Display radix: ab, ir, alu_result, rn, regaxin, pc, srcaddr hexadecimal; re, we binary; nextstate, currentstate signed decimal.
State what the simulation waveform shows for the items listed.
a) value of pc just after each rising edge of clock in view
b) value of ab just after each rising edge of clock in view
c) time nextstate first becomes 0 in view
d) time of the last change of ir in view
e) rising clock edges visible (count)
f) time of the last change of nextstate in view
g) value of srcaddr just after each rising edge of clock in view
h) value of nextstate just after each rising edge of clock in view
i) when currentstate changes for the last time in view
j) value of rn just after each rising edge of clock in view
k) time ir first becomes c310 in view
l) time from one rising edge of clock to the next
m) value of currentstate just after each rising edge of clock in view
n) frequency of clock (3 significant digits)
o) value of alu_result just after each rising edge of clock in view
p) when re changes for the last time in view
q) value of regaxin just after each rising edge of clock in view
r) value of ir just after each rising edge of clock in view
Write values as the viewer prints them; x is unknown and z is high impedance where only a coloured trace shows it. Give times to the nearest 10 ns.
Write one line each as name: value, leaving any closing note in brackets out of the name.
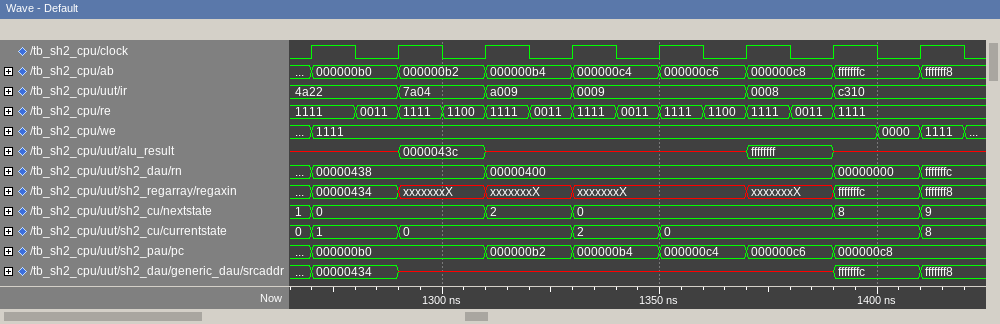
value of pc just after each rising edge of clock in view: 000000b0, 000000b0, 000000b2, 000000b4, 000000c4, 000000c6, 000000c8, 000000c8
value of ab just after each rising edge of clock in view: 000000b0, 000000b2, 000000b4, 000000c4, 000000c6, 000000c8, fffffffc, fffffff8
time nextstate first becomes 0 in view: 1270 ns
time of the last change of ir in view: 1390 ns
rising clock edges visible: 8
time of the last change of nextstate in view: 1410 ns
value of srcaddr just after each rising edge of clock in view: 00000434, x, x, x, x, x, fffffffc, fffffff8
value of nextstate just after each rising edge of clock in view: 0, 0, 2, 0, 0, 0, 8, 9
when currentstate changes for the last time in view: 1410 ns
value of rn just after each rising edge of clock in view: 00000438, 00000438, 00000400, 00000400, 00000400, 00000400, 00000000, fffffffc
time ir first becomes c310 in view: 1390 ns
time from one rising edge of clock to the next: 20 ns
value of currentstate just after each rising edge of clock in view: 1, 0, 0, 2, 0, 0, 0, 8
frequency of clock: 50.0 MHz
value of alu_result just after each rising edge of clock in view: x, 0000043c, x, x, x, ffffffff, x, x
when re changes for the last time in view: 1390 ns
value of regaxin just after each rising edge of clock in view: 00000434, xxxxxxxX, xxxxxxxX, xxxxxxxX, xxxxxxxX, xxxxxxxX, fffffffc, fffffff8
value of ir just after each rising edge of clock in view: 4a22, 7a04, a009, 0009, 0009, 0008, c310, c310
